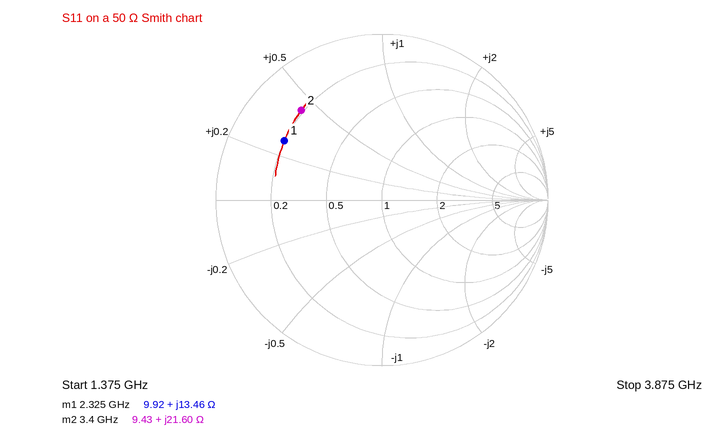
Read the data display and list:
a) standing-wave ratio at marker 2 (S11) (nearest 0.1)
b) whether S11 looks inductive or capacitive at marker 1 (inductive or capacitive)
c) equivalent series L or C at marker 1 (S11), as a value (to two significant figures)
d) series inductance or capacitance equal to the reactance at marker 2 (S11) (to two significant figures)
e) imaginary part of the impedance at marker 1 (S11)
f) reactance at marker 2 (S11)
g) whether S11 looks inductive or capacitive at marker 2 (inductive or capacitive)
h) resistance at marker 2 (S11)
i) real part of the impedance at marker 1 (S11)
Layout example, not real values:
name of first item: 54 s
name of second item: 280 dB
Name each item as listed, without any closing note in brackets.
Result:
standing-wave ratio at marker 2 (S11): 6.3
whether S11 looks inductive or capacitive at marker 1: inductive
equivalent series L or C at marker 1 (S11), as a value: 920 pH
series inductance or capacitance equal to the reactance at marker 2 (S11): 1.0 nH
imaginary part of the impedance at marker 1: +13.46 Ω
reactance at marker 2: +21.60 Ω
whether S11 looks inductive or capacitive at marker 2: inductive
resistance at marker 2: 9.43 Ω
real part of the impedance at marker 1: 9.92 Ω
